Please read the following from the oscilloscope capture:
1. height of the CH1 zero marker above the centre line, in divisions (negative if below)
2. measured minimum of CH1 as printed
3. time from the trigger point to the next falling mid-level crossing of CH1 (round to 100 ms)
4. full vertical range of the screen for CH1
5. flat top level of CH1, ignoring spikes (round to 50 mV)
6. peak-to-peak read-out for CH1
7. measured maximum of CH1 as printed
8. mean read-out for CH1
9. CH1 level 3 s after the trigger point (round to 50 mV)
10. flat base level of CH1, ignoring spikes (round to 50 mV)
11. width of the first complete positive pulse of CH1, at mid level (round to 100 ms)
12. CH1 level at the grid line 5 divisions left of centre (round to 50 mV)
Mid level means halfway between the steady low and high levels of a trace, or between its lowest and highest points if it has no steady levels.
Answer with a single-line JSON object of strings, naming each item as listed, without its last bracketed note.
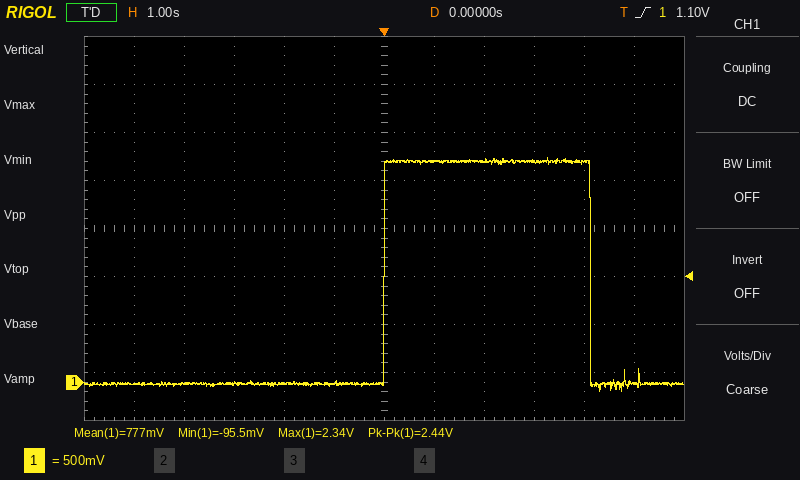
{"height of the CH1 zero marker above the centre line, in divisions": "-3.2 div", "measured minimum of CH1 as printed": "-95.5 mV", "time from the trigger point to the next falling mid-level crossing of CH1": "4.1 s", "full vertical range of the screen for CH1": "4 V", "flat top level of CH1, ignoring spikes": "2.30 V", "peak-to-peak read-out for CH1": "2.44 V", "measured maximum of CH1 as printed": "2.34 V", "mean read-out for CH1": "777 mV", "CH1 level 3 s after the trigger point": "2.30 V", "flat base level of CH1, ignoring spikes": "0 mV", "width of the first complete positive pulse of CH1, at mid level": "4.1 s", "CH1 level at the grid line 5 divisions left of centre": "0 mV"}
